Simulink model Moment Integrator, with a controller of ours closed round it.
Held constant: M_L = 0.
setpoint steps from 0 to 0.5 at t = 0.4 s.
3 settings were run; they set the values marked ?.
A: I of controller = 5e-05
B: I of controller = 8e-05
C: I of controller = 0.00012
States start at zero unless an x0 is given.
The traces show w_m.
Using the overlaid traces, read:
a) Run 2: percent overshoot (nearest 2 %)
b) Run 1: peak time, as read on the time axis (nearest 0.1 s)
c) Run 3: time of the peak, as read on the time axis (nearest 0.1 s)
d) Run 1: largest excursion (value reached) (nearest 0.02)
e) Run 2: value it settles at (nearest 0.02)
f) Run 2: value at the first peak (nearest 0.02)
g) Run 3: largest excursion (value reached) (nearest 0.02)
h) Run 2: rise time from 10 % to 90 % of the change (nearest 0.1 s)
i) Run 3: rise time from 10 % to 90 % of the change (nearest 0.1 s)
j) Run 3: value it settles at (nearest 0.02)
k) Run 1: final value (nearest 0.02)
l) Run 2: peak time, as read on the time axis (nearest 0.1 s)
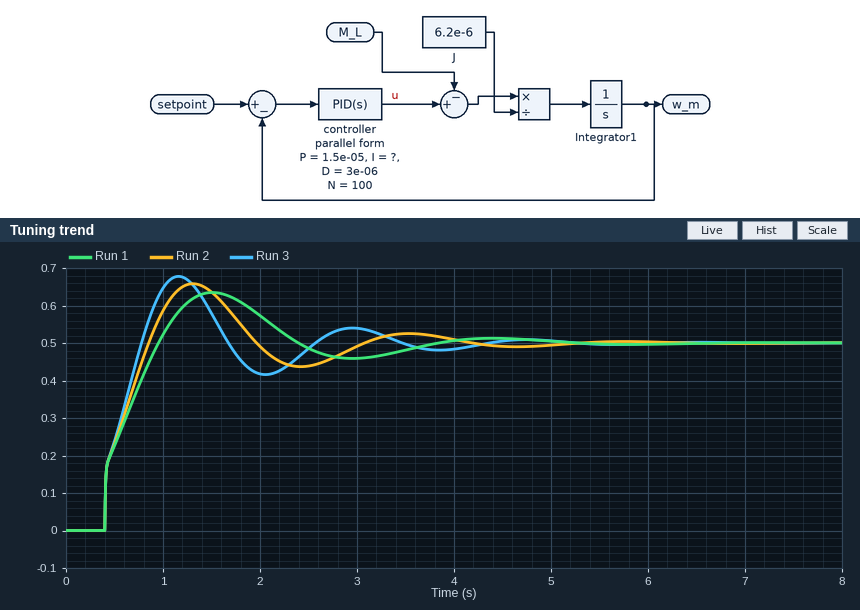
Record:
32 %
1.5 s
1.2 s
0.64
0.50
0.66
0.68
0.4 s
0.3 s
0.50
0.50
1.3 s
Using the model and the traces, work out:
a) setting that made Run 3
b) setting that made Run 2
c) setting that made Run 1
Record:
C
B
A
